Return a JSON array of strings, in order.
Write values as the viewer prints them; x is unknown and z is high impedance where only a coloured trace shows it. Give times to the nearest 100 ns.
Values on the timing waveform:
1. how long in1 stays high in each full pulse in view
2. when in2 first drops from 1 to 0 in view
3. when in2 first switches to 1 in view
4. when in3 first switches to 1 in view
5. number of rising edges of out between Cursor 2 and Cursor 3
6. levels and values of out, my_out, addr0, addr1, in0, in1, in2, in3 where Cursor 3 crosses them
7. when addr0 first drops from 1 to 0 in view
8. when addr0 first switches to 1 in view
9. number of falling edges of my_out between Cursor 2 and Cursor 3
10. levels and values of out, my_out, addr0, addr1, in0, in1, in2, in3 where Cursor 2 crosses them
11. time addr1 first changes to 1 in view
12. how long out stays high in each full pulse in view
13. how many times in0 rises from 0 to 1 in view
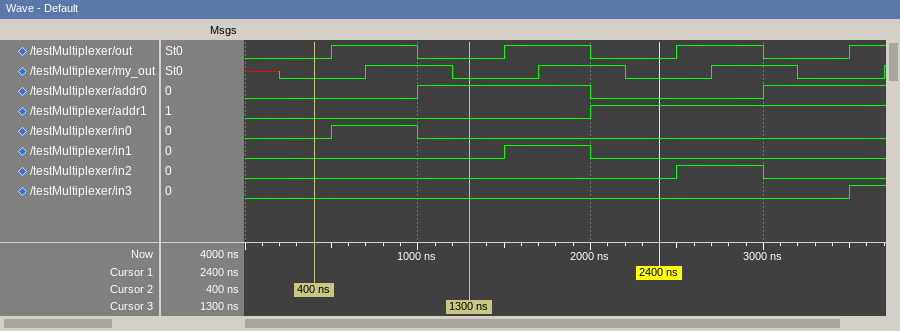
["500 ns", "3000 ns", "2500 ns", "3500 ns", "1", "out=0, my_out=0, addr0=1, addr1=0, in0=0, in1=0, in2=0, in3=0", "2000 ns", "1000 ns", "1", "out=0, my_out=0, addr0=0, addr1=0, in0=0, in1=0, in2=0, in3=0", "2000 ns", "500 ns, 500 ns, 500 ns", "1"]
